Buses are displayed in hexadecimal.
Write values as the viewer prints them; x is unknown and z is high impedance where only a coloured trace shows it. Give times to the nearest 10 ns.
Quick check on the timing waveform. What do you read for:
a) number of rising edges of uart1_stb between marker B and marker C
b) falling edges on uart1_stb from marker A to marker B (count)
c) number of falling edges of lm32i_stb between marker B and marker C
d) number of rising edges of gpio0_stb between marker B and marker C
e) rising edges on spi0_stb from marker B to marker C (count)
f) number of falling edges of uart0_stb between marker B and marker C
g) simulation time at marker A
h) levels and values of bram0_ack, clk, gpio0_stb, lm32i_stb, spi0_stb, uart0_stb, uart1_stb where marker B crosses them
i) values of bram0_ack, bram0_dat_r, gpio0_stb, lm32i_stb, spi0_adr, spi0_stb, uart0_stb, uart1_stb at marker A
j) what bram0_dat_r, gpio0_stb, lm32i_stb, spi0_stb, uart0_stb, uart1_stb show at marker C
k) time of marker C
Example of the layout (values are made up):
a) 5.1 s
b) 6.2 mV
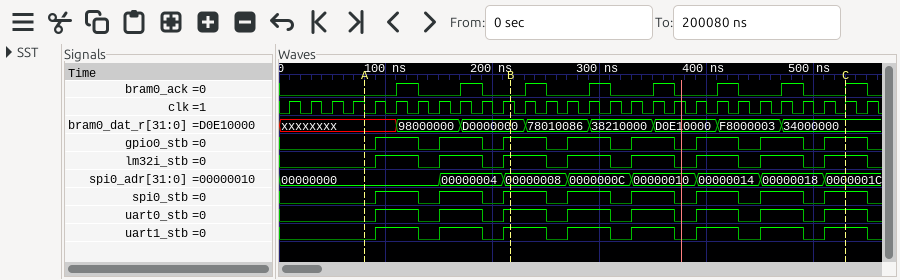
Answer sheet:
a) 5
b) 2
c) 5
d) 5
e) 5
f) 5
g) 80 ns
h) bram0_ack=0, clk=1, gpio0_stb=1, lm32i_stb=1, spi0_stb=1, uart0_stb=1, uart1_stb=1
i) bram0_ack=0, bram0_dat_r=xxxxxxxx, gpio0_stb=0, lm32i_stb=0, spi0_adr=00000000, spi0_stb=0, uart0_stb=0, uart1_stb=0
j) bram0_dat_r=34000000, gpio0_stb=1, lm32i_stb=1, spi0_stb=1, uart0_stb=1, uart1_stb=1
k) 530 ns
